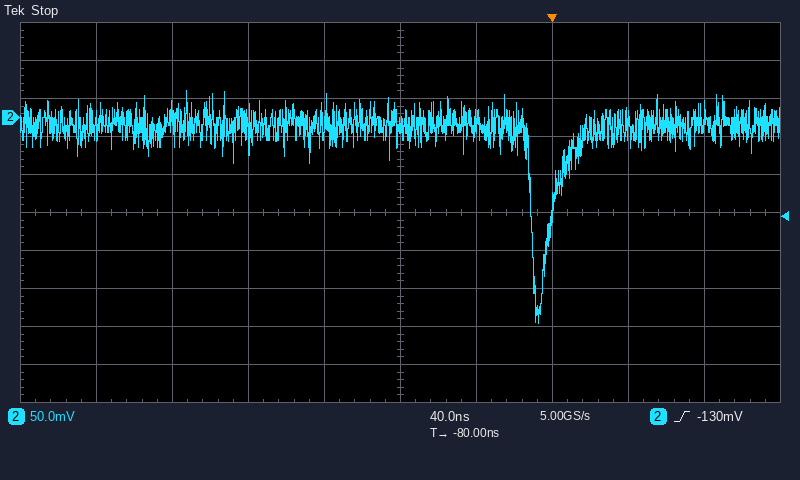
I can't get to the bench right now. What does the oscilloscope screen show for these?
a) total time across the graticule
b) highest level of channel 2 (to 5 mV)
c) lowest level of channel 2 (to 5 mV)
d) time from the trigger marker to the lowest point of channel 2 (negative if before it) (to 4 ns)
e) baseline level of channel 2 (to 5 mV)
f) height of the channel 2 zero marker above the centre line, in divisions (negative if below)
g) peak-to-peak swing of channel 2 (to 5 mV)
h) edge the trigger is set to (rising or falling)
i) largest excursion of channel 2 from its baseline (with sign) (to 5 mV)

400 ns
35 mV
-270 mV
-8 ns
-10 mV
+2.5 div
305 mV
rising
-260 mV
